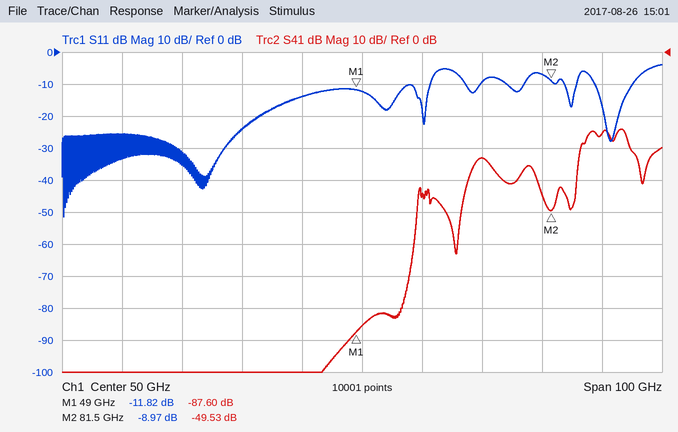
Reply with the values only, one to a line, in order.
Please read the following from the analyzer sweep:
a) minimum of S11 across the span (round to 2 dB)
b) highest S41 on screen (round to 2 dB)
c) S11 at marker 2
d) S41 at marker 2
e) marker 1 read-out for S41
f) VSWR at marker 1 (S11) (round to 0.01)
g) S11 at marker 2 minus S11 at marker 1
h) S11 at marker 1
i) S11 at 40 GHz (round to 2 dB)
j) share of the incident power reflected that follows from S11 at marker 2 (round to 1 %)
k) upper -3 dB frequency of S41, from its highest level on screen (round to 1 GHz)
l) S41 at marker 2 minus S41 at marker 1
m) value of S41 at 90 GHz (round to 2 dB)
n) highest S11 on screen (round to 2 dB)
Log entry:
-52 dB
-24 dB
-8.97 dB
-49.53 dB
-87.60 dB
1.69
2.85 dB
-11.82 dB
-14 dB
13 %
94 GHz
38.07 dB
-26 dB
-4 dB
